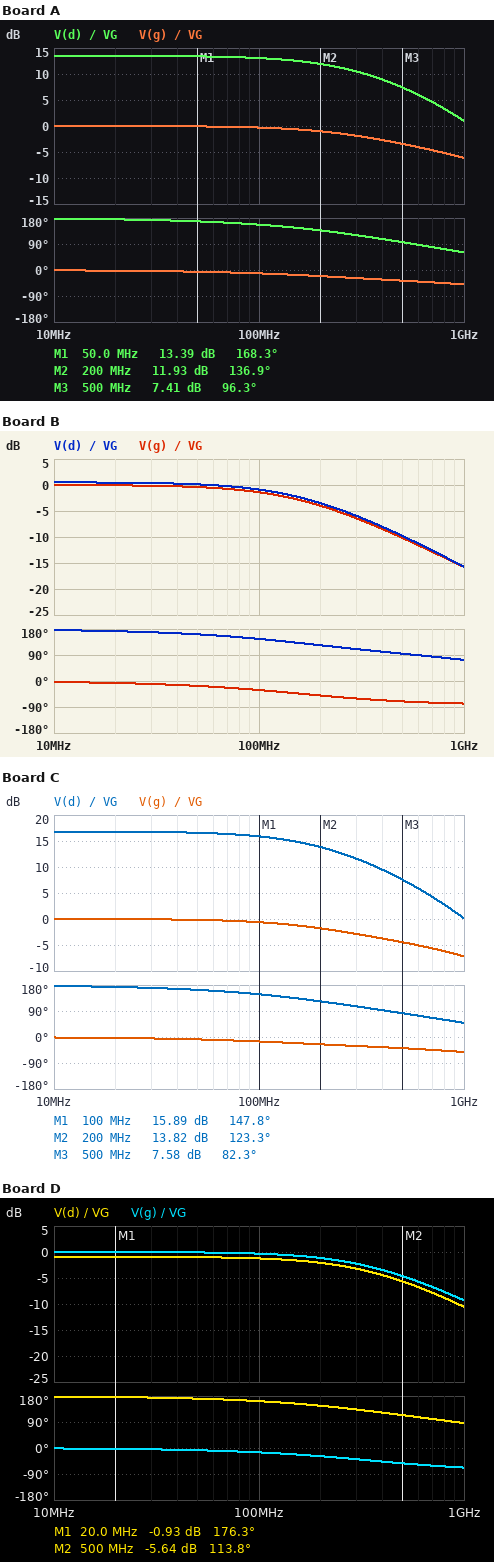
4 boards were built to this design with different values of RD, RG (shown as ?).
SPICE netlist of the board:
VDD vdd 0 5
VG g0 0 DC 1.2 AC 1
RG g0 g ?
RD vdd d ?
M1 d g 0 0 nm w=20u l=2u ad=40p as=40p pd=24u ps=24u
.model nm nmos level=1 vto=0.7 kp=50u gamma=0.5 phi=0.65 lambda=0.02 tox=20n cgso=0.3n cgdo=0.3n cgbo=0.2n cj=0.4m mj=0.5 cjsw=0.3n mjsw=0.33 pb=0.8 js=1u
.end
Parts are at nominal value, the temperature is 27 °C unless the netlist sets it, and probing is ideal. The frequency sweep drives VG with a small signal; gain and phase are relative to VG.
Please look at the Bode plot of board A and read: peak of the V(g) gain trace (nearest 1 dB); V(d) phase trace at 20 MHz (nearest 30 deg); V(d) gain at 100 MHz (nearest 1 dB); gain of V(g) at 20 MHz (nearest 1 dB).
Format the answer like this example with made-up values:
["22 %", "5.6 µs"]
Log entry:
["0 dB", "180 deg", "13 dB", "0 dB"]
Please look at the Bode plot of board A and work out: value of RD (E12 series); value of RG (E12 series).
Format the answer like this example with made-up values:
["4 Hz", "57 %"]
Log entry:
["18 kΩ", "3.9 kΩ"]
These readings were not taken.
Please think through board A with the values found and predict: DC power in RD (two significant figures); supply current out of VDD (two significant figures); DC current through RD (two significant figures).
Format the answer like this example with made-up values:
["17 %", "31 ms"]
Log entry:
["81 µW", "67 µA", "67 µA"]
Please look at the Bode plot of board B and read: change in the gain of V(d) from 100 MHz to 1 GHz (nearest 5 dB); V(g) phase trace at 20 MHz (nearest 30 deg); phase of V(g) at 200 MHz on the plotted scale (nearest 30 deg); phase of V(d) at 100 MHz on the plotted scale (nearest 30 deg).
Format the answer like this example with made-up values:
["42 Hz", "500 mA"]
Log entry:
["-15 dB", "0 deg", "-60 deg", "150 deg"]
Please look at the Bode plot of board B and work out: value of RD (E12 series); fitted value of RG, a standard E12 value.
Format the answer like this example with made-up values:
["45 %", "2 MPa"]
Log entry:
["3.9 kΩ", "15 kΩ"]
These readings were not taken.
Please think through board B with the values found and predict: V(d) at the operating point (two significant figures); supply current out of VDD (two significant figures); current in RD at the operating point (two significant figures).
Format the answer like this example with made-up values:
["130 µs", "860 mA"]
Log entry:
["4.7 V", "68 µA", "68 µA"]
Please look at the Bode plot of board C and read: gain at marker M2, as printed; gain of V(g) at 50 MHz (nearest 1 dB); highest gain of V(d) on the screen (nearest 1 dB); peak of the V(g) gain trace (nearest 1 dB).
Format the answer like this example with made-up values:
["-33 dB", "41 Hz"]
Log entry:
["13.82 dB", "0 dB", "17 dB", "0 dB"]
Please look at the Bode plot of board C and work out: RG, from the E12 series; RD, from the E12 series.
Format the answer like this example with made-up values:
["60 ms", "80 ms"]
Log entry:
["4.7 kΩ", "27 kΩ"]
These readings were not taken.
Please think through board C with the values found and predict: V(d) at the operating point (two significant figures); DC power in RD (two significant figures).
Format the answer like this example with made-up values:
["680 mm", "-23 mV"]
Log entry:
["3.2 V", "120 µW"]
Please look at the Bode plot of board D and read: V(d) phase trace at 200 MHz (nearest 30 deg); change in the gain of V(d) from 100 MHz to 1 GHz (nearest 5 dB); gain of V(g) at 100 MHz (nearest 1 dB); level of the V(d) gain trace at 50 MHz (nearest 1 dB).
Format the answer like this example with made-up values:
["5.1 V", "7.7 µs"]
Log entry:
["150 deg", "-10 dB", "0 dB", "-1 dB"]
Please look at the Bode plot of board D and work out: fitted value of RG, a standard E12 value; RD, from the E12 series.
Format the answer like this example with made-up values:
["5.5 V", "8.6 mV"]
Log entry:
["6.8 kΩ", "3.3 kΩ"]
